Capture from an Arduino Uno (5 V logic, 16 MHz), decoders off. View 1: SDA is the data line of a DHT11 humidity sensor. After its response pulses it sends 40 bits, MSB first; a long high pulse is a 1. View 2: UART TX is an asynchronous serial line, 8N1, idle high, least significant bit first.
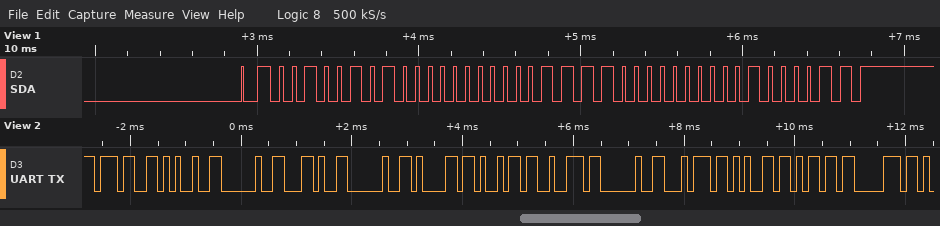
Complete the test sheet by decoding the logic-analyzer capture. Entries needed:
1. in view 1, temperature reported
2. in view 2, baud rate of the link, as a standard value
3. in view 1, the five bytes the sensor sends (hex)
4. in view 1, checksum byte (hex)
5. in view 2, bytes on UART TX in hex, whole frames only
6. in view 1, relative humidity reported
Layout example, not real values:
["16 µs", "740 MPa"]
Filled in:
["30.0 °C", "9600 baud", "25 00 1E 00 43", "0x43", "37 25 20 2C 20 61 69 72 20 74 65 6D 70", "37 %"]
